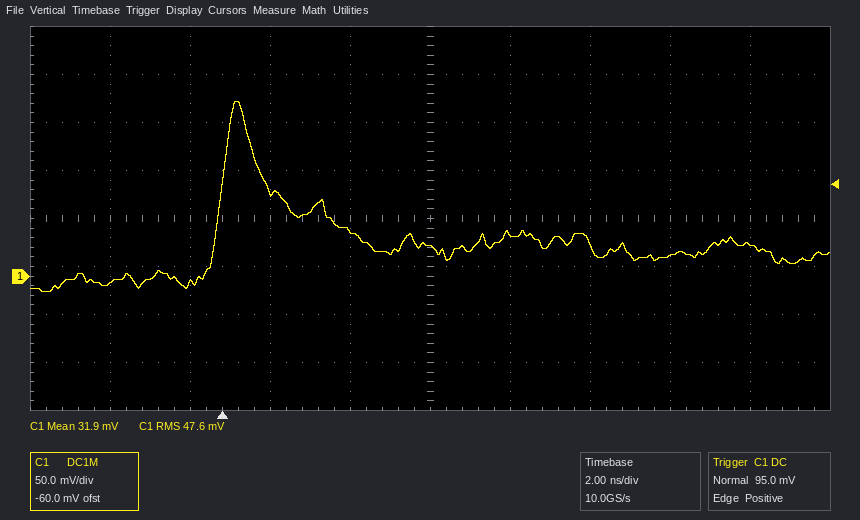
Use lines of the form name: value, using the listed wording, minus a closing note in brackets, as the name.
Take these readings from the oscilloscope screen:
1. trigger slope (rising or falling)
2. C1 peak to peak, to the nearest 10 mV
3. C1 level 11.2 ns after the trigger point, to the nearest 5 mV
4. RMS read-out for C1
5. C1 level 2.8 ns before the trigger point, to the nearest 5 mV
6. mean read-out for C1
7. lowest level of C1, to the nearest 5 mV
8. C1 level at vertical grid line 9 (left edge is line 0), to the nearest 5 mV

trigger slope: rising
C1 peak to peak, to the nearest 10 mV: 200 mV
C1 level 11.2 ns after the trigger point, to the nearest 5 mV: 20 mV
RMS read-out for C1: 47.6 mV
C1 level 2.8 ns before the trigger point, to the nearest 5 mV: -5 mV
mean read-out for C1: 31.9 mV
lowest level of C1, to the nearest 5 mV: -15 mV
C1 level at vertical grid line 9 (left edge is line 0), to the nearest 5 mV: 35 mV
